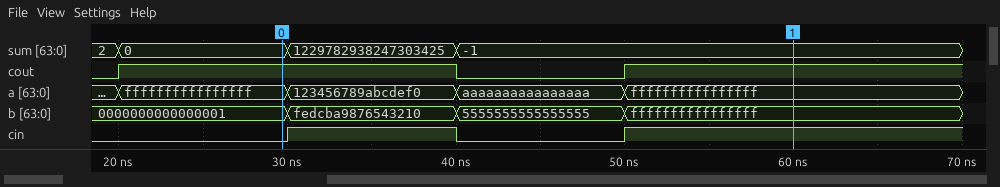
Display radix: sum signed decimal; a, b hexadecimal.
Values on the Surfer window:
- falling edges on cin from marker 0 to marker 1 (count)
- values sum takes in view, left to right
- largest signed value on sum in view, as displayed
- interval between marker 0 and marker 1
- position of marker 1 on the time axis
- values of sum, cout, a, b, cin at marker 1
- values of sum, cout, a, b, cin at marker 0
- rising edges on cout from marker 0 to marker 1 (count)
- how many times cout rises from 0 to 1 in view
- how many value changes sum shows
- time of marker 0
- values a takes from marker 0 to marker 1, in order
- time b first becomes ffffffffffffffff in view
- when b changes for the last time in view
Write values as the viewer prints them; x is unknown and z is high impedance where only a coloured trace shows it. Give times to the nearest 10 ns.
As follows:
1
2, 0, 1229782938247303425, -1
1229782938247303425
30 ns
60 ns
sum=-1, cout=1, a=ffffffffffffffff, b=ffffffffffffffff, cin=1
sum=0, cout=1, a=ffffffffffffffff, b=0000000000000001, cin=0
1
2
3
30 ns
ffffffffffffffff, 123456789abcdef0, aaaaaaaaaaaaaaaa, ffffffffffffffff
50 ns
50 ns
